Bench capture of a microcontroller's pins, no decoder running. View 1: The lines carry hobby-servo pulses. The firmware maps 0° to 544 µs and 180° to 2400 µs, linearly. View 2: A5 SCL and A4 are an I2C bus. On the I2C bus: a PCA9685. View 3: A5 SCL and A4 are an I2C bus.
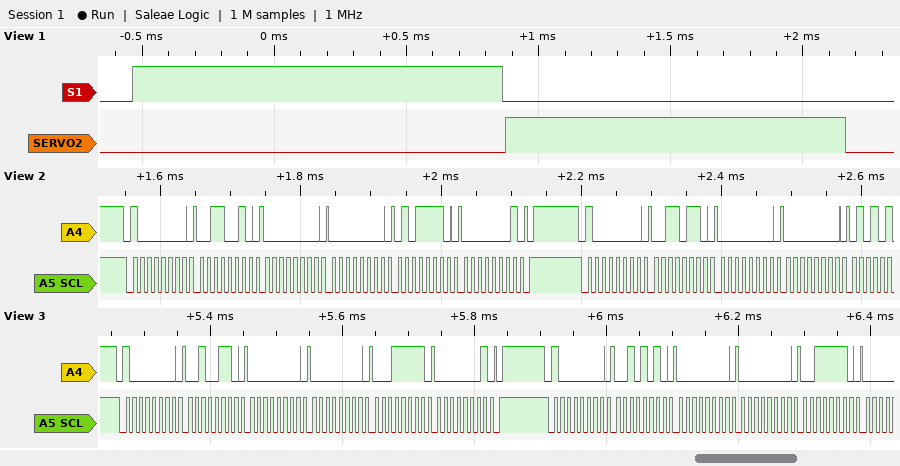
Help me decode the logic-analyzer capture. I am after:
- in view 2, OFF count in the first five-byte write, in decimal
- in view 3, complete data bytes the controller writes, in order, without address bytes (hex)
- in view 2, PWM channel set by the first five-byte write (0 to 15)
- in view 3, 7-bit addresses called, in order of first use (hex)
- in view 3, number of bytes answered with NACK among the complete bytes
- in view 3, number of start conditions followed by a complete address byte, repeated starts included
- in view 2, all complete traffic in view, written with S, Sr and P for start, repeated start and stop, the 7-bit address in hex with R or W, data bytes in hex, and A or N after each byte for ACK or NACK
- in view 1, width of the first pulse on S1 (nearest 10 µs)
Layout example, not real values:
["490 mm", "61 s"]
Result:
["350", "26 00 00 1F 01 2A 00 00 3E", "11", "0x40", "0", "2", "S 40W A 32 A 00 A 00 A 5E A 01 A P S 40W A 36 A 00 A 00 A", "1400 µs"]
